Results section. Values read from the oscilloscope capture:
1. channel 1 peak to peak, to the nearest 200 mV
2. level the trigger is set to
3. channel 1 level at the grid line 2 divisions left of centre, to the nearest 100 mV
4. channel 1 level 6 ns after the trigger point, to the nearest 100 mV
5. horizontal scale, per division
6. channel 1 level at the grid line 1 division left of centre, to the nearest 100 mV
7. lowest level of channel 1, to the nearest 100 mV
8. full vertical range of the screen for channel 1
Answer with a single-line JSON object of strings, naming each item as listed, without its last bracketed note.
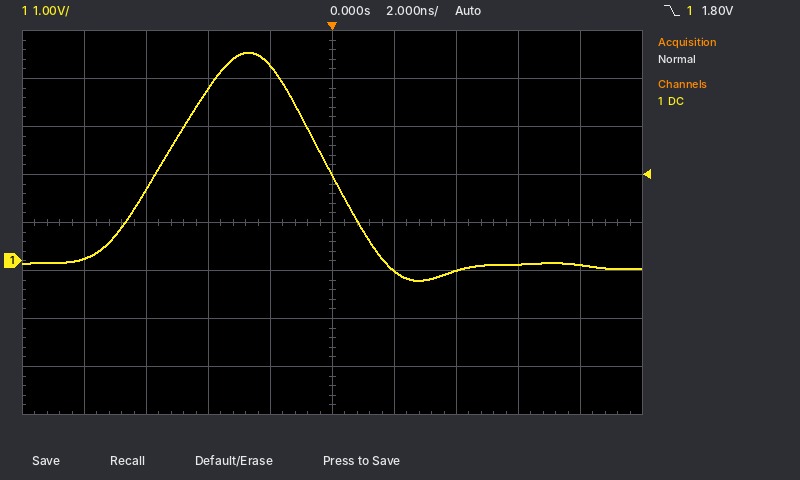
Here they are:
{"channel 1 peak to peak, to the nearest 200 mV": "4.8 V", "level the trigger is set to": "1.80 V", "channel 1 level at the grid line 2 divisions left of centre, to the nearest 100 mV": "3.6 V", "channel 1 level 6 ns after the trigger point, to the nearest 100 mV": "-100 mV", "horizontal scale, per division": "2 ns", "channel 1 level at the grid line 1 division left of centre, to the nearest 100 mV": "4.1 V", "lowest level of channel 1, to the nearest 100 mV": "-400 mV", "full vertical range of the screen for channel 1": "8 V"}
